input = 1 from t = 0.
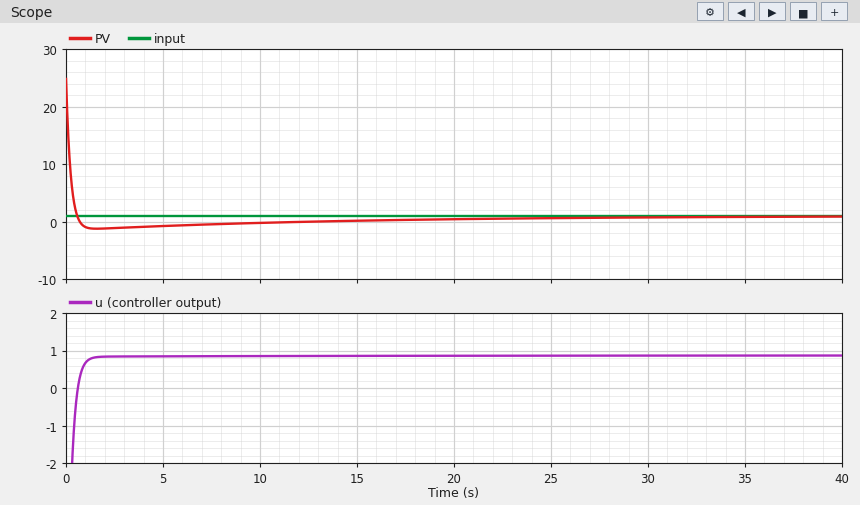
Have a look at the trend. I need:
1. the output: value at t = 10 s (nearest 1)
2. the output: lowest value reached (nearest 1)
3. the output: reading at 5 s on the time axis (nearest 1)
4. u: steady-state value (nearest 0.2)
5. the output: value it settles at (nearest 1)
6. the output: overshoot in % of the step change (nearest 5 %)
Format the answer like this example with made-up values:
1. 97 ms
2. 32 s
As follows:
1. 0
2. -1
3. -1
4. 0.8
5. 1
6. 10 %
